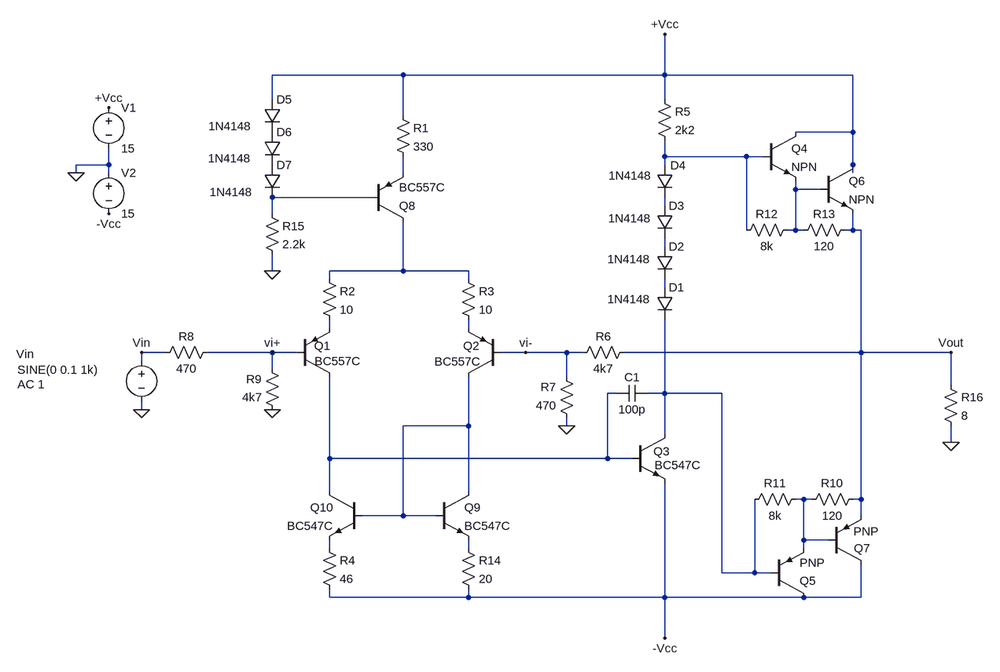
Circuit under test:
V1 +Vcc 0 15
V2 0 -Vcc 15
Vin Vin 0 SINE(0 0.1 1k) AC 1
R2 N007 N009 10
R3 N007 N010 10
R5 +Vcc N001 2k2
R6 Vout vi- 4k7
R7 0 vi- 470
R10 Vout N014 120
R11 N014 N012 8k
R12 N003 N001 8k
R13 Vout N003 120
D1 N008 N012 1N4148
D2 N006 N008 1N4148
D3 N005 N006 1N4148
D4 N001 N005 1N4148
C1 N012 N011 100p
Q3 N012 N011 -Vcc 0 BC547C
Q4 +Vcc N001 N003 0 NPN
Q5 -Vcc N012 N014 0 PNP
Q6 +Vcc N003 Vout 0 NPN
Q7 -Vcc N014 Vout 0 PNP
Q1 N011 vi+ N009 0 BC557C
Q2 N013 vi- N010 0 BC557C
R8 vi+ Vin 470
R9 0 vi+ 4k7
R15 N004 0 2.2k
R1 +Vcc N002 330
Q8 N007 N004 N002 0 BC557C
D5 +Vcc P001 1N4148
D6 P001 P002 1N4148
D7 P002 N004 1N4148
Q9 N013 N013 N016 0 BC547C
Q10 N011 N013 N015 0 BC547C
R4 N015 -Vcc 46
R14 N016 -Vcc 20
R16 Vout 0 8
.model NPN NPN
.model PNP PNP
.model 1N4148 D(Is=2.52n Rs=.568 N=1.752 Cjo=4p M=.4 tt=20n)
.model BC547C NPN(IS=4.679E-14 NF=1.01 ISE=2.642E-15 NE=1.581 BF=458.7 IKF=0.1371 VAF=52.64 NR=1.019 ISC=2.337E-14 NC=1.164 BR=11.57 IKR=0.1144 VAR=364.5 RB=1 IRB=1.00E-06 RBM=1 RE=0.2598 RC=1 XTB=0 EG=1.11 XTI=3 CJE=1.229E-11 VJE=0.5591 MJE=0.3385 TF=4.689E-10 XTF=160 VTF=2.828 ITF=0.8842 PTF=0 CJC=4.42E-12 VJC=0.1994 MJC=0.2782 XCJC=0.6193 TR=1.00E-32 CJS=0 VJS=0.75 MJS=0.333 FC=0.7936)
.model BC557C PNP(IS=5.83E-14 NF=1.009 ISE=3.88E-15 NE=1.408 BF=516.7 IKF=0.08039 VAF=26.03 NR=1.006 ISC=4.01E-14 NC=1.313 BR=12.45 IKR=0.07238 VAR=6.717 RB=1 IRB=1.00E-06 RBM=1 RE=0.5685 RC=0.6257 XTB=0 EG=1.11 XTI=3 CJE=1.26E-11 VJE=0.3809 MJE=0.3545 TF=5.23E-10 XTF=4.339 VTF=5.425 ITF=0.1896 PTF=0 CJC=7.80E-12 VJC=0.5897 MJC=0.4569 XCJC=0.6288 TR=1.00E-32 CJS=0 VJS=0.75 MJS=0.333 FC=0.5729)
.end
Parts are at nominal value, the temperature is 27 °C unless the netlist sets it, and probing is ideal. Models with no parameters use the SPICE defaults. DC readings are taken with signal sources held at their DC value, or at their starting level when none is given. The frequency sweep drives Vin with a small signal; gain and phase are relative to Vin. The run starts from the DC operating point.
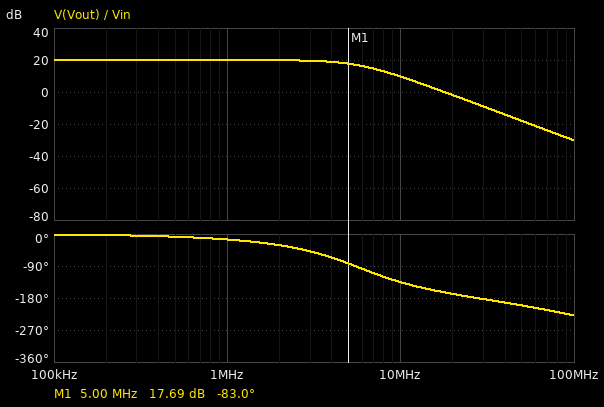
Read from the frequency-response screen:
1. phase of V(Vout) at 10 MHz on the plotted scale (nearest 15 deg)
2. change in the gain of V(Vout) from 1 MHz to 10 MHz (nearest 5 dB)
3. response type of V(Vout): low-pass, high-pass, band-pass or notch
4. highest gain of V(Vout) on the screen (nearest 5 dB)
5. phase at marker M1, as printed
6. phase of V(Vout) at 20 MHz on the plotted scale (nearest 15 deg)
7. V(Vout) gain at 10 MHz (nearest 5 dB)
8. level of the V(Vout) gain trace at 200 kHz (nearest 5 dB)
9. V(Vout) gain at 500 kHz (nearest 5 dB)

-135 deg
-10 dB
low-pass
20 dB
-83.0 deg
-165 deg
10 dB
20 dB
20 dB
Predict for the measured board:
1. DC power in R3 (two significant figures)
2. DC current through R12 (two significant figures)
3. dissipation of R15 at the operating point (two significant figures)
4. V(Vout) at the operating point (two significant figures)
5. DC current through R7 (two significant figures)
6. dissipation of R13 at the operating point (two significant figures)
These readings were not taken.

69 µW
98 µA
77 mW
-310 mV
56 µA
370 µW
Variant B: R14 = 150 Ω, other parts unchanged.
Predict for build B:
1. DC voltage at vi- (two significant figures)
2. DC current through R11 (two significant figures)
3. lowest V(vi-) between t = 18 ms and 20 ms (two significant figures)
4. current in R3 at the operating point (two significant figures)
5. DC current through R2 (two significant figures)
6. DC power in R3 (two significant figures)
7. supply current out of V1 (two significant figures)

48 mV
98 µA
-43 mV
1.1 mA
3.0 mA
12 µW
83 mA
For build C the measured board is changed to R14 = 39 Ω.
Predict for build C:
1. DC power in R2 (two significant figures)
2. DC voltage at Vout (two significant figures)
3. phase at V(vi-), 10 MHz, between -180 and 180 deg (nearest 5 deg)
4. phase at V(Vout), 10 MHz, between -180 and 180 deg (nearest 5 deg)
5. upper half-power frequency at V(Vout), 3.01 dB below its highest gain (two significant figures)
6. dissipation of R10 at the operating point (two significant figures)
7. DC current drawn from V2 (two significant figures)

37 µW
-68 mV
50 deg
-140 deg
4.4 MHz
5.5 mW
21 mA
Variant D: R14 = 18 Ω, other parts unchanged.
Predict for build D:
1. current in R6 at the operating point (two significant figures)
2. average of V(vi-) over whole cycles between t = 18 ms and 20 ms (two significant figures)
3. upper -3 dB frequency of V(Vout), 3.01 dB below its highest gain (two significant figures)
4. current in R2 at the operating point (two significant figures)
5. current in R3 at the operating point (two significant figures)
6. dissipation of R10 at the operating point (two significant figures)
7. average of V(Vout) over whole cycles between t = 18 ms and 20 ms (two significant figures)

66 µA
-29 mV
5.3 MHz
1.4 mA
2.7 mA
6.3 mW
-340 mV
